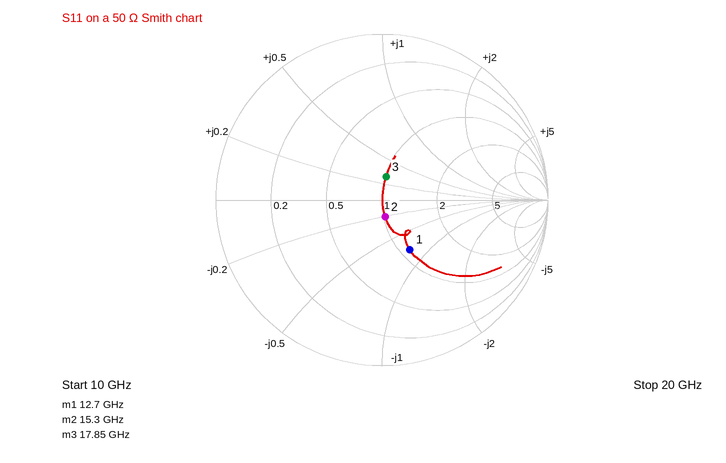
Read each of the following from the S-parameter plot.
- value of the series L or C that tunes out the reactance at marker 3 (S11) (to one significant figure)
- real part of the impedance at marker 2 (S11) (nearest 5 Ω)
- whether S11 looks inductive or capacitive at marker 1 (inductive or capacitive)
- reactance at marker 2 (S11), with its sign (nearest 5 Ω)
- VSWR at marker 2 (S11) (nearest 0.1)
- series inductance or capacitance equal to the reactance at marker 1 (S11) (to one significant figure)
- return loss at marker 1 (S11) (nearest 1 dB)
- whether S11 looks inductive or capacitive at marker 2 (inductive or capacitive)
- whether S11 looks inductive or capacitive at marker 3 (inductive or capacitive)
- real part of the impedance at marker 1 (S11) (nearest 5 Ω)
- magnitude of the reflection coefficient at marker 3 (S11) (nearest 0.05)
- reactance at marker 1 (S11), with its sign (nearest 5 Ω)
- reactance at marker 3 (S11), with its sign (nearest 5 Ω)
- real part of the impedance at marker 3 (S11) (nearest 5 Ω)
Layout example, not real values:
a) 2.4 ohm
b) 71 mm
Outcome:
a) 600 fF
b) 50 Ω
c) capacitive
d) -10 Ω
e) 1.2
f) 300 fF
g) 9 dB
h) capacitive
i) inductive
j) 55 Ω
k) 0.15
l) -40 Ω
m) +15 Ω
n) 50 Ω
